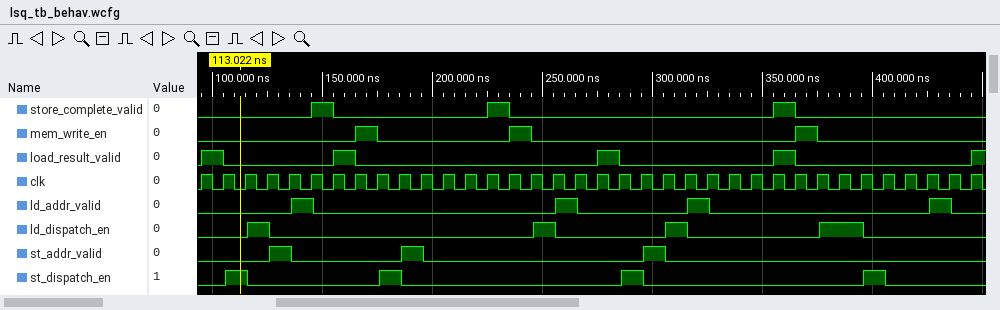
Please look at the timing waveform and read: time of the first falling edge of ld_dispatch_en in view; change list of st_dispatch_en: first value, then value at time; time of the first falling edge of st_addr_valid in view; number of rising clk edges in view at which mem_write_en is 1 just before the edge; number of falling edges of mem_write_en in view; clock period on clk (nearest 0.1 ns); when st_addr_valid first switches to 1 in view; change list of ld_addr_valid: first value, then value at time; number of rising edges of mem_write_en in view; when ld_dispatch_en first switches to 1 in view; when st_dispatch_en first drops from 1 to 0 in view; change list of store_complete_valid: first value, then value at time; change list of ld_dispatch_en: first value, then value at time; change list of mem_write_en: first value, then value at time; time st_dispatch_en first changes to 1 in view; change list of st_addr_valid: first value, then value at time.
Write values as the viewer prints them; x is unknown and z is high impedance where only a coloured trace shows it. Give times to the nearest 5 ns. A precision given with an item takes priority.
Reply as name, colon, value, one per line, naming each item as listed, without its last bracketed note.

time of the first falling edge of ld_dispatch_en in view: 125 ns
change list of st_dispatch_en: first value, then value at time: 0, 1 at 105 ns, 0 at 115 ns, 1 at 175 ns, 0 at 185 ns, 1 at 285 ns, 0 at 295 ns, 1 at 395 ns, 0 at 405 ns
time of the first falling edge of st_addr_valid in view: 135 ns
number of rising clk edges in view at which mem_write_en is 1 just before the edge: 3
number of falling edges of mem_write_en in view: 3
clock period on clk: 10 ns
when st_addr_valid first switches to 1 in view: 125 ns
change list of ld_addr_valid: first value, then value at time: 0, 1 at 135 ns, 0 at 145 ns, 1 at 255 ns, 0 at 265 ns, 1 at 315 ns, 0 at 325 ns, 1 at 425 ns, 0 at 435 ns
number of rising edges of mem_write_en in view: 3
when ld_dispatch_en first switches to 1 in view: 115 ns
when st_dispatch_en first drops from 1 to 0 in view: 115 ns
change list of store_complete_valid: first value, then value at time: 0, 1 at 145 ns, 0 at 155 ns, 1 at 225 ns, 0 at 235 ns, 1 at 355 ns, 0 at 365 ns
change list of ld_dispatch_en: first value, then value at time: 0, 1 at 115 ns, 0 at 125 ns, 1 at 245 ns, 0 at 255 ns, 1 at 305 ns, 0 at 315 ns, 1 at 375 ns, 0 at 395 ns
change list of mem_write_en: first value, then value at time: 0, 1 at 165 ns, 0 at 175 ns, 1 at 235 ns, 0 at 245 ns, 1 at 365 ns, 0 at 375 ns
time st_dispatch_en first changes to 1 in view: 105 ns
change list of st_addr_valid: first value, then value at time: 0, 1 at 125 ns, 0 at 135 ns, 1 at 185 ns, 0 at 195 ns, 1 at 295 ns, 0 at 305 ns
